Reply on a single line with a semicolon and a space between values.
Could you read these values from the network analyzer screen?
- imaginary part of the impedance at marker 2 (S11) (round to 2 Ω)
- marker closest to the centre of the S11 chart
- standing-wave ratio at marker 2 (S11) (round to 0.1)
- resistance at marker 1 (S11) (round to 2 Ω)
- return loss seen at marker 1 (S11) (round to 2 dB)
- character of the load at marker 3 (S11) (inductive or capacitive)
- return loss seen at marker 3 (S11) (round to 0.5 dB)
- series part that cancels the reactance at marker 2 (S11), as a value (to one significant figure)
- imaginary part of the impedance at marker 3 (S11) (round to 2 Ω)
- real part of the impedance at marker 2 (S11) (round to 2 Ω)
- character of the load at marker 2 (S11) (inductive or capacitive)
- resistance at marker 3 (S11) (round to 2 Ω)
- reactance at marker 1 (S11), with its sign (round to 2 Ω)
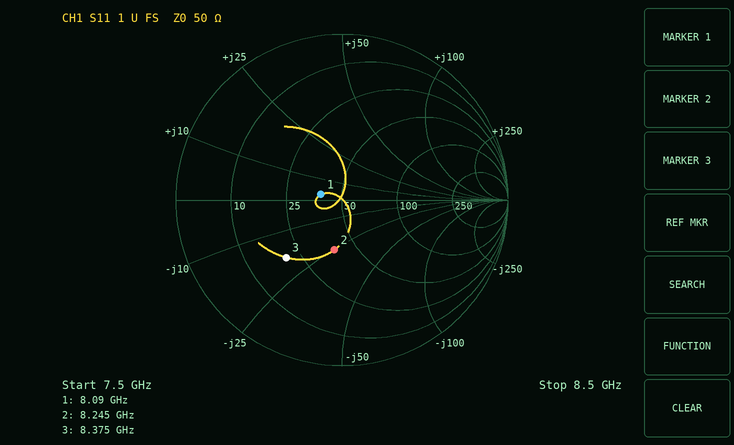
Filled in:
-26 Ω; marker 1; 1.9; 38 Ω; 18 dB; capacitive; 6.5 dB; 500 pH; -18 Ω; 38 Ω; capacitive; 20 Ω; +2 Ω
